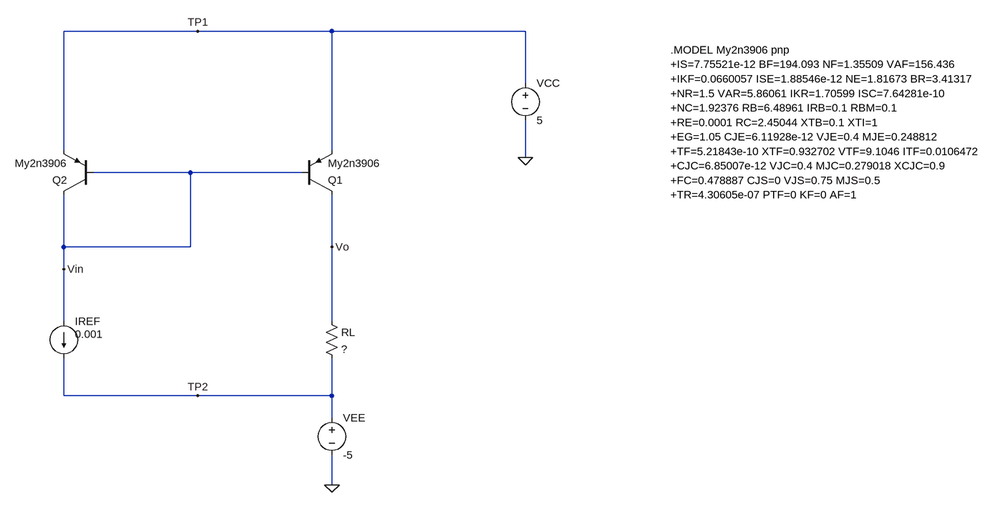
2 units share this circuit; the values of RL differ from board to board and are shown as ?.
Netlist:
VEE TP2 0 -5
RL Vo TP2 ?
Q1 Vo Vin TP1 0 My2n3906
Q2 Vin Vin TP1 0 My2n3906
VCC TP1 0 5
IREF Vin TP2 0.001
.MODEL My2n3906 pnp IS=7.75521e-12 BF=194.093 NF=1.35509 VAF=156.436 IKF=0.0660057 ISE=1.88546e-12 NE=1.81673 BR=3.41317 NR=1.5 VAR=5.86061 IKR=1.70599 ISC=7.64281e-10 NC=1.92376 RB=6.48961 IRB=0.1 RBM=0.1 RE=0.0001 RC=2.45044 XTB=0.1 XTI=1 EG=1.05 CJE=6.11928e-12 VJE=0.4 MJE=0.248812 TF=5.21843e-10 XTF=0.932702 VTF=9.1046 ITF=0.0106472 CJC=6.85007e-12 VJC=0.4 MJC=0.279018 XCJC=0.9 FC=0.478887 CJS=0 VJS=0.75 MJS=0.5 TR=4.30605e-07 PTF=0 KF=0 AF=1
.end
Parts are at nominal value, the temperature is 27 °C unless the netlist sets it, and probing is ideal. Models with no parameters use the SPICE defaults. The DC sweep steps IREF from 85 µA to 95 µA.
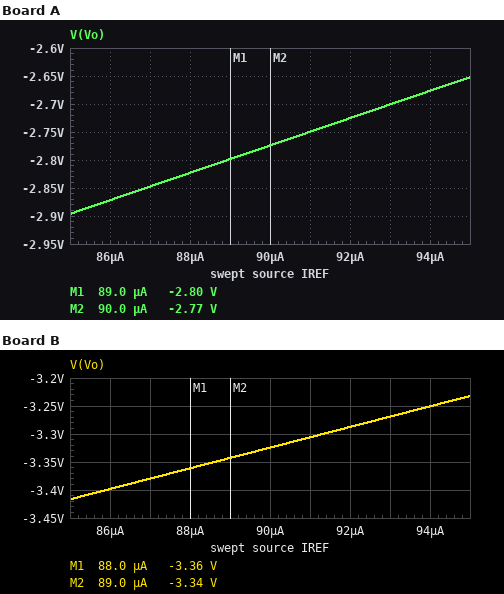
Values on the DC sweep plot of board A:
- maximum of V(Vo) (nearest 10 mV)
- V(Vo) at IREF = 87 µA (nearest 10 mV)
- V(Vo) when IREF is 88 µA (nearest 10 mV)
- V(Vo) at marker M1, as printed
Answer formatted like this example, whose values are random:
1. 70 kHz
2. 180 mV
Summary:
1. -2.65 V
2. -2.85 V
3. -2.82 V
4. -2.80 V
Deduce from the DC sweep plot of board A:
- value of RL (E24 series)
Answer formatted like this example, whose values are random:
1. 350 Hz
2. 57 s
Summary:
1. 24 kΩ
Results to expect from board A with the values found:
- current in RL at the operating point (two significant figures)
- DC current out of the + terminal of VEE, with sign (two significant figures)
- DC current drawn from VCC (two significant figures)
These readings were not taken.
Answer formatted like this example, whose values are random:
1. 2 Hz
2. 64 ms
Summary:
1. 420 µA
2. -1.4 mA
3. 1.4 mA
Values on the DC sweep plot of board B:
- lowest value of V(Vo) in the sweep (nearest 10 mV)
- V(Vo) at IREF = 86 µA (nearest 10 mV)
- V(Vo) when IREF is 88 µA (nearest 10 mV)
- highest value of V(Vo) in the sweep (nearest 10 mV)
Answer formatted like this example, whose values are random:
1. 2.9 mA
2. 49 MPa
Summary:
1. -3.42 V
2. -3.40 V
3. -3.36 V
4. -3.23 V
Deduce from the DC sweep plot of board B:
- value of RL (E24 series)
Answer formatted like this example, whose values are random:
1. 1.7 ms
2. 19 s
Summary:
1. 18 kΩ
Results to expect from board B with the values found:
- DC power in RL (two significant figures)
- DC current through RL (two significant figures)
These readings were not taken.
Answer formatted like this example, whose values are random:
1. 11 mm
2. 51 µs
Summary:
1. 5.5 mW
2. 550 µA
